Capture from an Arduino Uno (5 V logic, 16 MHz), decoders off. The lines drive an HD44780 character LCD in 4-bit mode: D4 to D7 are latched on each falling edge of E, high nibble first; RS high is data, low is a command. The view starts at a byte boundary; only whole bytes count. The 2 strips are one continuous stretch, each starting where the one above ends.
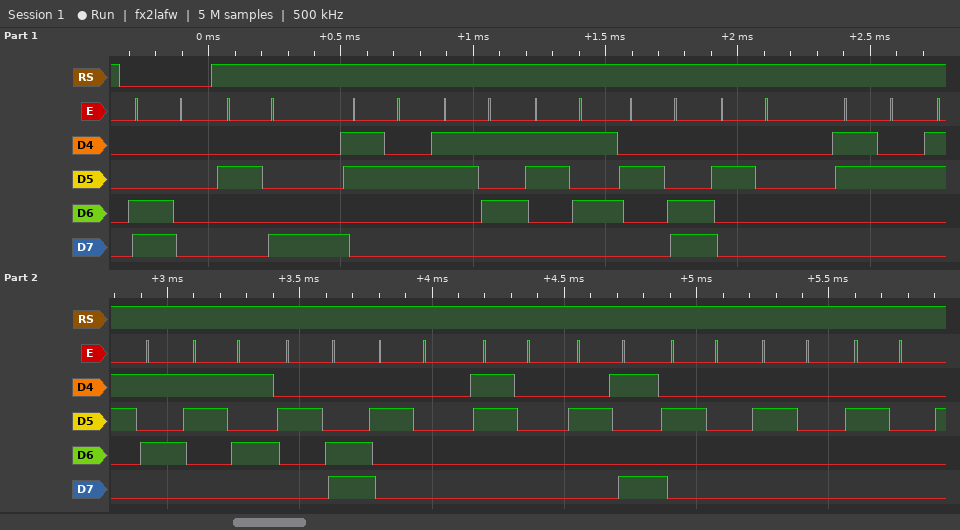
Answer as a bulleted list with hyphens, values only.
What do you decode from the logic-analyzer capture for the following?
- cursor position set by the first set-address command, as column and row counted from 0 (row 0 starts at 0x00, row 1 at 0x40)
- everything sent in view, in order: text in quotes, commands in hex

- column 0, row 1
- 0xC0 "(255, 255, 0)   "
